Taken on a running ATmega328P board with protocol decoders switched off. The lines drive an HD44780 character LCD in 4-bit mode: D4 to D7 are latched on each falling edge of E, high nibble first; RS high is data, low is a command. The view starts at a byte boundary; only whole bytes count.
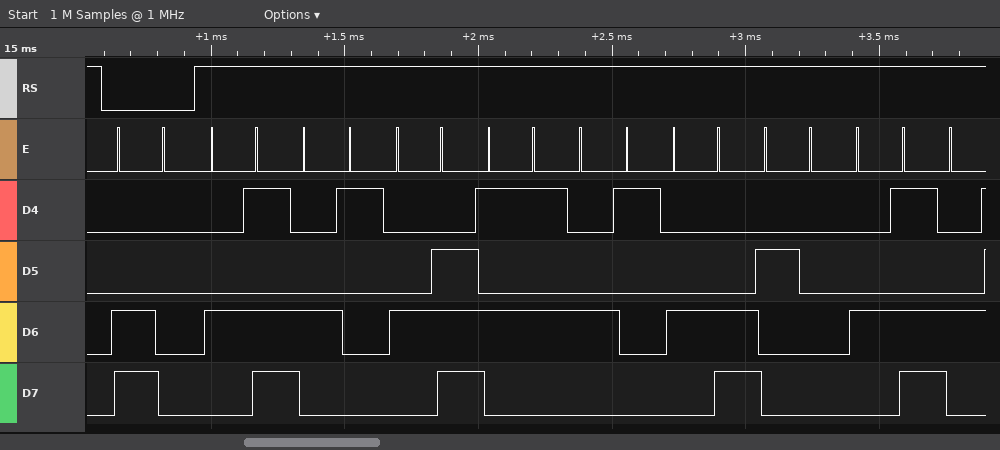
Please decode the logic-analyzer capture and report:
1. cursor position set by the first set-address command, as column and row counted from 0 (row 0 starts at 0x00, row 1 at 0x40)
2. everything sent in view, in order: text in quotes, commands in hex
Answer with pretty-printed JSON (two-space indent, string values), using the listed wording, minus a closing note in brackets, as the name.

{
  "cursor position set by the first set-address command, as column and row counted from 0": "column 0, row 1",
  "everything sent in view, in order: text in quotes, commands in hex": "0xC0 \"MANUAL M\""
}
